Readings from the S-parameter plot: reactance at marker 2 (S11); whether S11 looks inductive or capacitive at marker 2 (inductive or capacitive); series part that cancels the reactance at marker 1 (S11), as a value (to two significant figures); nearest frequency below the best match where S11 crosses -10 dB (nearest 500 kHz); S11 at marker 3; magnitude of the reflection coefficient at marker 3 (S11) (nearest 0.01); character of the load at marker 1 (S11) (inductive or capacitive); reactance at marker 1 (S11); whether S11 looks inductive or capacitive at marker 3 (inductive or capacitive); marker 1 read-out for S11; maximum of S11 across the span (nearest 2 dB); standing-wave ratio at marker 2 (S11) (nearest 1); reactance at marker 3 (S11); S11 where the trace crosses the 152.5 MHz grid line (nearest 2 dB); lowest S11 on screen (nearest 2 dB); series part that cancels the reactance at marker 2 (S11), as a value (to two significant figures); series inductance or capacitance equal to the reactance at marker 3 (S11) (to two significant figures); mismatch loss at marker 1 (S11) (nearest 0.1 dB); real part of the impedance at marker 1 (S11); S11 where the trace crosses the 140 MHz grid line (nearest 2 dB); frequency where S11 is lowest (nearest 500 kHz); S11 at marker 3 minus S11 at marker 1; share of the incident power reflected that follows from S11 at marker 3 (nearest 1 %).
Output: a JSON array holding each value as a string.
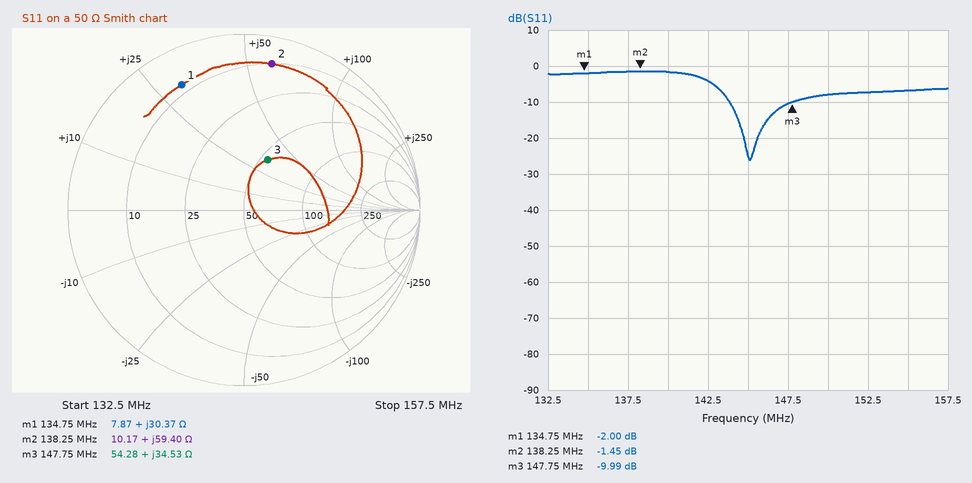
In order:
["+59.40 Ω", "inductive", "39 pF", "144.0 MHz", "-9.99 dB", "0.32", "inductive", "+30.37 Ω", "inductive", "-2.00 dB", "-2 dB", "12", "+34.53 Ω", "-8 dB", "-26 dB", "19 pF", "37 nH", "4.3 dB", "7.87 Ω", "-2 dB", "145.0 MHz", "-7.99 dB", "10 %"]
